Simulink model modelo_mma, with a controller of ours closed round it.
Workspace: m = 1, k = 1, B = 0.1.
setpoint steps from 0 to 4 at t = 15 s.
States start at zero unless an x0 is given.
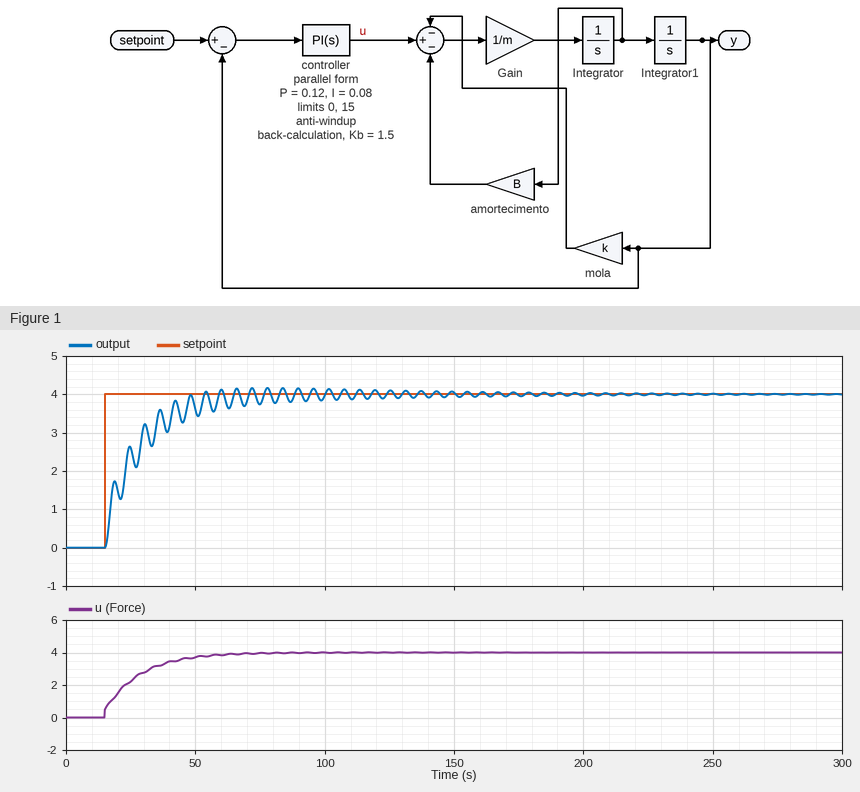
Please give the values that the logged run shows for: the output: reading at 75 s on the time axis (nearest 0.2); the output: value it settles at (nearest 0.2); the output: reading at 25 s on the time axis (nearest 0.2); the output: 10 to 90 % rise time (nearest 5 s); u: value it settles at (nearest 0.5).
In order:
3.8
4.0
2.6
25 s
4.0
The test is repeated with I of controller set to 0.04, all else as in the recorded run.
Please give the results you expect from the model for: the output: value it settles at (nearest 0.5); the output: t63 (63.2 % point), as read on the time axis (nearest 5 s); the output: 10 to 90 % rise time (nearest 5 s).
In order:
4.0
35 s
55 s
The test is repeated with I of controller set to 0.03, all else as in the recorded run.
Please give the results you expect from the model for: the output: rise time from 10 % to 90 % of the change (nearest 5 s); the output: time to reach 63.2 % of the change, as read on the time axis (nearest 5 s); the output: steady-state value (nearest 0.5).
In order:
80 s
45 s
4.0
